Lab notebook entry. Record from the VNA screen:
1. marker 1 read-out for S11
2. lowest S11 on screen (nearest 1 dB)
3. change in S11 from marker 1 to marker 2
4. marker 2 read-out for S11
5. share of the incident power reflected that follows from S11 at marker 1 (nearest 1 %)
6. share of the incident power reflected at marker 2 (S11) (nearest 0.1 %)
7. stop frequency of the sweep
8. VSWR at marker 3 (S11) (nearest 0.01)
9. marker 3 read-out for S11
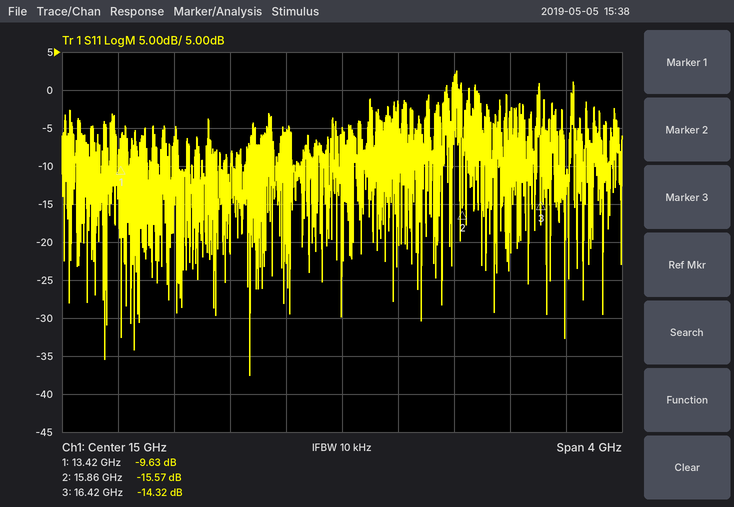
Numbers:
-9.63 dB
-38 dB
-5.94 dB
-15.57 dB
11 %
2.8 %
17 GHz
1.48
-14.32 dB
